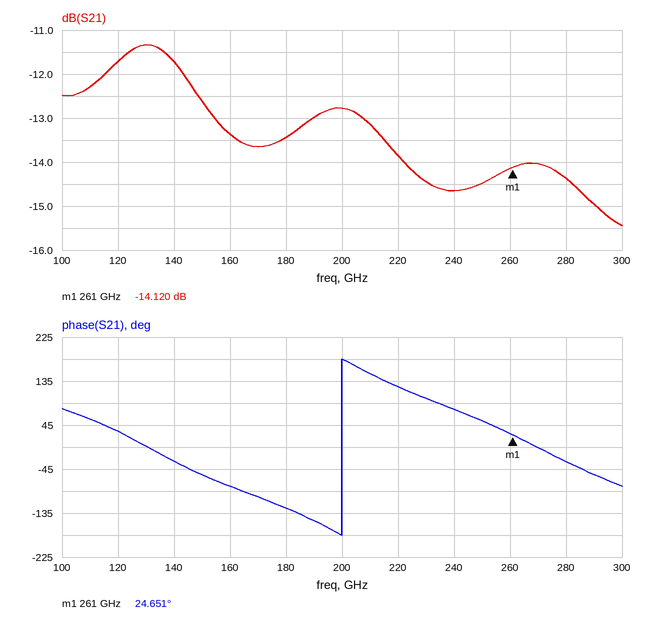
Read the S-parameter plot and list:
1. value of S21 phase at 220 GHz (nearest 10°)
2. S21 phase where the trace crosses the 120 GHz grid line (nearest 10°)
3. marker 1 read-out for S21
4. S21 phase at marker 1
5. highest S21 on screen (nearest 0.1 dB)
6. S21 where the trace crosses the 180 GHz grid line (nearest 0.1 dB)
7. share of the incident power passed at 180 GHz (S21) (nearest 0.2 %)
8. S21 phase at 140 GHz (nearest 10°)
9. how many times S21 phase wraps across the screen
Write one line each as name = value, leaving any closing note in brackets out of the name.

value of S21 phase at 220 GHz = 120°
S21 phase where the trace crosses the 120 GHz grid line = 30°
marker 1 read-out for S21 = -14.120 dB
S21 phase at marker 1 = 24.651°
highest S21 on screen = -11.3 dB
S21 where the trace crosses the 180 GHz grid line = -13.4 dB
share of the incident power passed at 180 GHz (S21) = 4.6 %
S21 phase at 140 GHz = -30°
how many times S21 phase wraps across the screen = 1
